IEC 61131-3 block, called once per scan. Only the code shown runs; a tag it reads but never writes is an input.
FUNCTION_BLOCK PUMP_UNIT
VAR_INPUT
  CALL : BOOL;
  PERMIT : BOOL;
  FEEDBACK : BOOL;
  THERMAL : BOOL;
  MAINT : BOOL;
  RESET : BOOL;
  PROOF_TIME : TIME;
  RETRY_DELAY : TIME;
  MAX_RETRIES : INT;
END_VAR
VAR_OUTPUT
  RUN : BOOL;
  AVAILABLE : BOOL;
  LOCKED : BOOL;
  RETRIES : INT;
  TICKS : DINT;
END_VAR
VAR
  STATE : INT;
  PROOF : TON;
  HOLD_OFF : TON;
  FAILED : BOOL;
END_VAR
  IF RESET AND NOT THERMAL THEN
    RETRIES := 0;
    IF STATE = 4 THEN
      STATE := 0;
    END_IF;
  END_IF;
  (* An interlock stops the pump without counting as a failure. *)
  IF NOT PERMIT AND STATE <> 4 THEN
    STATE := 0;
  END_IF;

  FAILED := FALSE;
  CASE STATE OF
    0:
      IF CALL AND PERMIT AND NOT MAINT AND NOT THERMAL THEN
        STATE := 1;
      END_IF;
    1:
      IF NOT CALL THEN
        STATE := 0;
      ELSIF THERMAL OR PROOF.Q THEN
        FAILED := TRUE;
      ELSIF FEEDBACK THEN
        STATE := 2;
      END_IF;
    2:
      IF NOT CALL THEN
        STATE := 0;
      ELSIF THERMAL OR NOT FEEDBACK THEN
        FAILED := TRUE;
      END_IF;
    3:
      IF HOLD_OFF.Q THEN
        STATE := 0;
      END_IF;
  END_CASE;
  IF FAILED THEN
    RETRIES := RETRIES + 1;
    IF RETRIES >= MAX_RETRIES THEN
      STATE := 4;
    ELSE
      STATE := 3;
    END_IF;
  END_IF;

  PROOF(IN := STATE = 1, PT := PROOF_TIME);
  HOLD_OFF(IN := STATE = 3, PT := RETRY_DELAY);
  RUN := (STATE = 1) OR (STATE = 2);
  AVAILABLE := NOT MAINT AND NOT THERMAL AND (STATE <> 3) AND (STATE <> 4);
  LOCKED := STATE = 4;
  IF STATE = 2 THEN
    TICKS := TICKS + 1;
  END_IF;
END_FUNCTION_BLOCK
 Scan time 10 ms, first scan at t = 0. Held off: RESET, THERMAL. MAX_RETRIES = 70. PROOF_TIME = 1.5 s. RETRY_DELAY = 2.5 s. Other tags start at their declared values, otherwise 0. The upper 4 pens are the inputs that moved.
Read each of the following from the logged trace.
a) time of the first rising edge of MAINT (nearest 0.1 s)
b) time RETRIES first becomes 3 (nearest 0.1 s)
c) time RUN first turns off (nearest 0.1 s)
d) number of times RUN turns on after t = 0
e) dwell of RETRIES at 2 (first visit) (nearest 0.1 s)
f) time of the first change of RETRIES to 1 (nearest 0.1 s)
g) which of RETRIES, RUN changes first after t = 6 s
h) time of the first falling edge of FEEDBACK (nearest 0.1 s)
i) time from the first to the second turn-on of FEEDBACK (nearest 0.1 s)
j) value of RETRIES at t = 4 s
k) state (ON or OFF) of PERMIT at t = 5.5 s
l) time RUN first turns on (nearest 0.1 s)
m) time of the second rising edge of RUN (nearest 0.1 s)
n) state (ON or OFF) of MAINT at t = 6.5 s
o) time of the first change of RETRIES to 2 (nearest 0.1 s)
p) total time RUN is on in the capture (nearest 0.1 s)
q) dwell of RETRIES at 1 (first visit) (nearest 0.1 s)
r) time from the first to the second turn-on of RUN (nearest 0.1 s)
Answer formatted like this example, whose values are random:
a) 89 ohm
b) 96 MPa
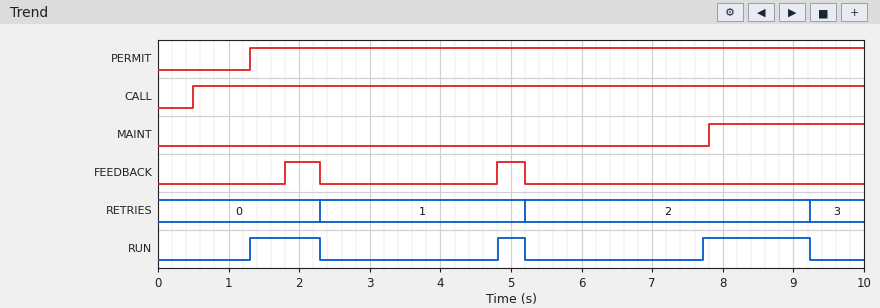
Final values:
a) 7.8 s
b) 9.2 s
c) 2.3 s
d) 3
e) 4.0 s
f) 2.3 s
g) RUN
h) 2.3 s
i) 3.0 s
j) 1
k) ON
l) 1.3 s
m) 4.8 s
n) OFF
o) 5.2 s
p) 2.9 s
q) 2.9 s
r) 3.5 s
